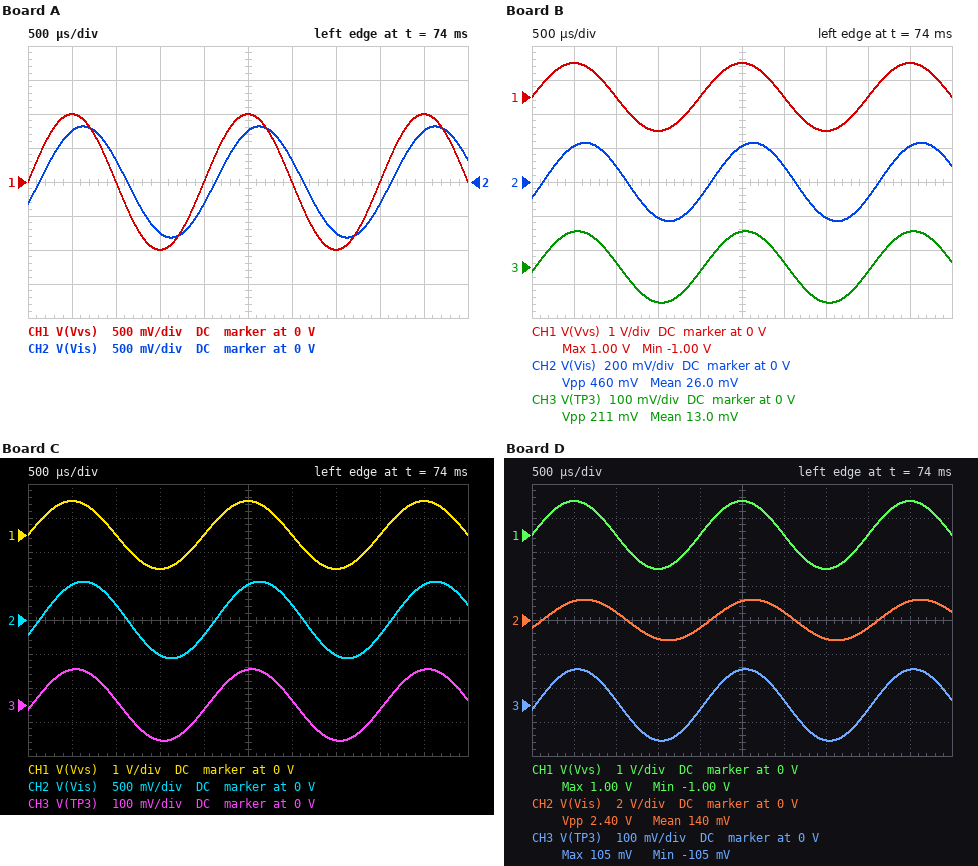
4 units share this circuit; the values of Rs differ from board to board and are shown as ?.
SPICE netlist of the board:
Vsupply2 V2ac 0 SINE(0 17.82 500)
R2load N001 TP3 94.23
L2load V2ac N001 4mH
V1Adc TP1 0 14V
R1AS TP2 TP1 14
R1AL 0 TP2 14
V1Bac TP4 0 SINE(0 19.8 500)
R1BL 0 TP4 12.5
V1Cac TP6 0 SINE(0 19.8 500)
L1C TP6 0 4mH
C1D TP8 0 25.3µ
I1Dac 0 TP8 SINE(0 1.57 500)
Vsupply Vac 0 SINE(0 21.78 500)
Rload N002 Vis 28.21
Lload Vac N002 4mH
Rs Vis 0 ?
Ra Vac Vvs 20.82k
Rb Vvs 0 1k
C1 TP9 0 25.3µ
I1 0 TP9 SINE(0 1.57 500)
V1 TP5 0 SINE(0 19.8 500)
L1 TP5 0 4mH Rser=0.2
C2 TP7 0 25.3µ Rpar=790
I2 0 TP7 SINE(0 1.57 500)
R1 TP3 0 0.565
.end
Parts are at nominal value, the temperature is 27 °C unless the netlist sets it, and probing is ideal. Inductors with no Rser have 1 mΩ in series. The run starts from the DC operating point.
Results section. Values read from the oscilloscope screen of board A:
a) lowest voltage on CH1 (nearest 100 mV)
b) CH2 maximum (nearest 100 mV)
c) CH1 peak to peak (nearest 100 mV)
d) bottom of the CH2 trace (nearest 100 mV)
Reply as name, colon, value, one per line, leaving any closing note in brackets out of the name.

lowest voltage on CH1: -1.0 V
CH2 maximum: 800 mV
CH1 peak to peak: 2.0 V
bottom of the CH2 trace: -800 mV
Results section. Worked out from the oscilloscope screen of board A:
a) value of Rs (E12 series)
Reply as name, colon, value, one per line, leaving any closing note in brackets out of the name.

value of Rs: 1.2 Ω
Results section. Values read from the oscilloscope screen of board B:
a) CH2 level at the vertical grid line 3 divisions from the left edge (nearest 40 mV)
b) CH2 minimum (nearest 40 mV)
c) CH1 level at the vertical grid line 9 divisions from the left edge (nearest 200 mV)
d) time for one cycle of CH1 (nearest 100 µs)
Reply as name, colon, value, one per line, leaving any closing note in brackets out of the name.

CH2 level at the vertical grid line 3 divisions from the left edge: -200 mV
CH2 minimum: -240 mV
CH1 level at the vertical grid line 9 divisions from the left edge: 1.0 V
time for one cycle of CH1: 2.0 ms
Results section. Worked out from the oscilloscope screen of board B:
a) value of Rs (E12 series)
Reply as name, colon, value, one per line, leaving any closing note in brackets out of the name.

value of Rs: 0.33 Ω
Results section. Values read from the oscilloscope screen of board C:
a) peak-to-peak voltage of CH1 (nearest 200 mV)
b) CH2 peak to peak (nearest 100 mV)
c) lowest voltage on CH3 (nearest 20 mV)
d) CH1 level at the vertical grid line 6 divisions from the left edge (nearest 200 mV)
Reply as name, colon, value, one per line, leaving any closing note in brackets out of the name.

peak-to-peak voltage of CH1: 2.0 V
CH2 peak to peak: 1.1 V
lowest voltage on CH3: -100 mV
CH1 level at the vertical grid line 6 divisions from the left edge: 0 V
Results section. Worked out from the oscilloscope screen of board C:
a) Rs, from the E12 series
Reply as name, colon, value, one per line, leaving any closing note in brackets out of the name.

Rs, from the E12 series: 0.82 Ω
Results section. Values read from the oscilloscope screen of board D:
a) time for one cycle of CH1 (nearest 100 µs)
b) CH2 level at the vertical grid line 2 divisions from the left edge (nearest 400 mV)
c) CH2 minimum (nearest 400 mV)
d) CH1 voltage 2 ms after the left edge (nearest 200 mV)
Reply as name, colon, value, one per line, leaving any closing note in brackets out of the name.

time for one cycle of CH1: 2.0 ms
CH2 level at the vertical grid line 2 divisions from the left edge: 400 mV
CH2 minimum: -1.2 V
CH1 voltage 2 ms after the left edge: 0 V
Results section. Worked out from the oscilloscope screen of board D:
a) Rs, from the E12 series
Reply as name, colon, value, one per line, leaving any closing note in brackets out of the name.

Rs, from the E12 series: 1.8 Ω
